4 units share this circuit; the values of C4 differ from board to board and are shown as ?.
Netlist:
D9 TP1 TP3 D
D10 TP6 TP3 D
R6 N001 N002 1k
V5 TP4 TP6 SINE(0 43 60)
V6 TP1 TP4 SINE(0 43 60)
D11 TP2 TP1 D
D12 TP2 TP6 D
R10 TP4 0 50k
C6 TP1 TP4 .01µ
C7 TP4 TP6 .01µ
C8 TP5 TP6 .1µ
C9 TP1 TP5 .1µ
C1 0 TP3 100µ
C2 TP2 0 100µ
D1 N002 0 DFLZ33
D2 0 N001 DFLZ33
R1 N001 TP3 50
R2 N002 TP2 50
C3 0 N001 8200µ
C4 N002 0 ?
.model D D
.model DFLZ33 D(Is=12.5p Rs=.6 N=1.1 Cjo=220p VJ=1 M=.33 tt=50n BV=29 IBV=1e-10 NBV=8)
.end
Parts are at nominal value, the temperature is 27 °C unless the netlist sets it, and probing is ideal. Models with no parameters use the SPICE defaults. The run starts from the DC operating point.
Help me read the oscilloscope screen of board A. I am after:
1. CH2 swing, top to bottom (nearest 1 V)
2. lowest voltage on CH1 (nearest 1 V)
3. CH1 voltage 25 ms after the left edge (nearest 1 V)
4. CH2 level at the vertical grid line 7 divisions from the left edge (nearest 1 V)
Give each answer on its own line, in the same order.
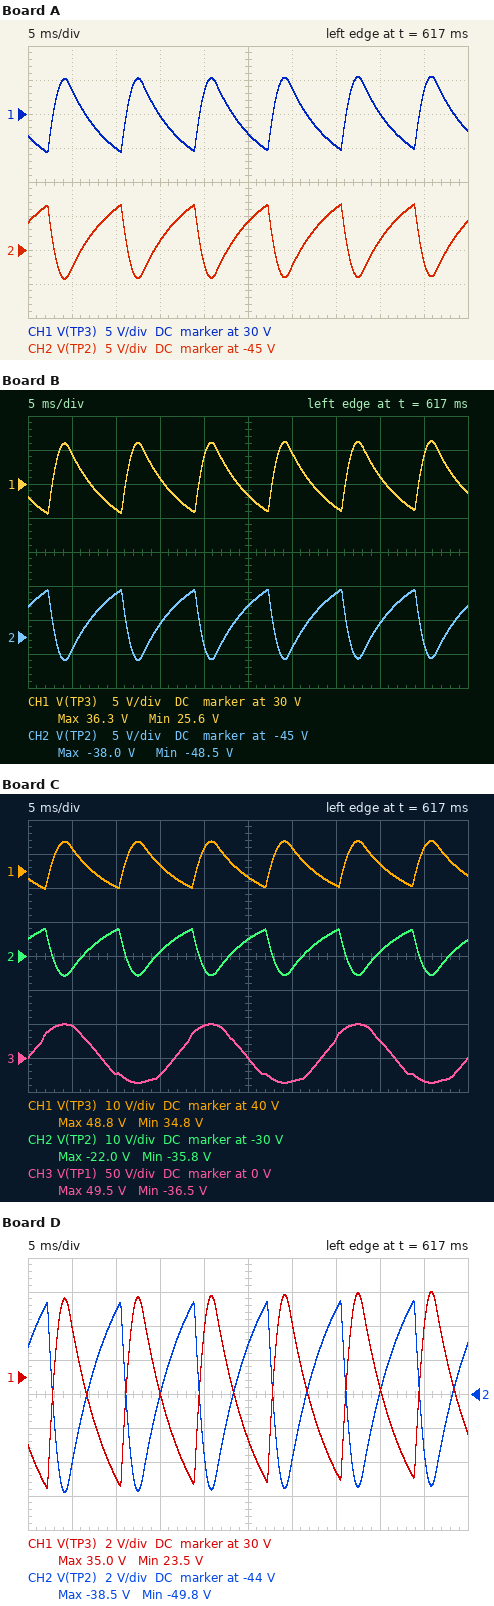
11 V
24 V
27 V
-39 V
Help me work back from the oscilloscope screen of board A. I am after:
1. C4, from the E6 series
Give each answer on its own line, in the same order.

3.3 mF
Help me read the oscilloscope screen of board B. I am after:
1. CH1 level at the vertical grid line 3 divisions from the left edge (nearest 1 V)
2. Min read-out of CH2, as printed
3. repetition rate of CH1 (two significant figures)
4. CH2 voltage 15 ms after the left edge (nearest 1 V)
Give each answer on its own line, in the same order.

31 V
-48.5 V
120 Hz
-43 V
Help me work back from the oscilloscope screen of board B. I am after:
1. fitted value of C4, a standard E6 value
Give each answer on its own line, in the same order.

4.7 mF
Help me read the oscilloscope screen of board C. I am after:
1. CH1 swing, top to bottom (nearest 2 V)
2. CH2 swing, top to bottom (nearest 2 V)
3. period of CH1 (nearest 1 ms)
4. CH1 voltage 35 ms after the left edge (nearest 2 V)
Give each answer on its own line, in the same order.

14 V
14 V
8 ms
36 V
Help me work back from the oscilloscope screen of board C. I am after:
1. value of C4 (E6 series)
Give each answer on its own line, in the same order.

15 mF
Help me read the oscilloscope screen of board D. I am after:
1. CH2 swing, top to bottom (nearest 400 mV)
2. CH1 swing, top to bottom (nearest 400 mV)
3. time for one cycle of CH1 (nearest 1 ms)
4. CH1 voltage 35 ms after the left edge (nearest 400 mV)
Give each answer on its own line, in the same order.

11.2 V
11.6 V
8 ms
24.4 V
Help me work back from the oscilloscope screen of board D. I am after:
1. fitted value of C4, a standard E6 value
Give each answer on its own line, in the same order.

2.2 mF
